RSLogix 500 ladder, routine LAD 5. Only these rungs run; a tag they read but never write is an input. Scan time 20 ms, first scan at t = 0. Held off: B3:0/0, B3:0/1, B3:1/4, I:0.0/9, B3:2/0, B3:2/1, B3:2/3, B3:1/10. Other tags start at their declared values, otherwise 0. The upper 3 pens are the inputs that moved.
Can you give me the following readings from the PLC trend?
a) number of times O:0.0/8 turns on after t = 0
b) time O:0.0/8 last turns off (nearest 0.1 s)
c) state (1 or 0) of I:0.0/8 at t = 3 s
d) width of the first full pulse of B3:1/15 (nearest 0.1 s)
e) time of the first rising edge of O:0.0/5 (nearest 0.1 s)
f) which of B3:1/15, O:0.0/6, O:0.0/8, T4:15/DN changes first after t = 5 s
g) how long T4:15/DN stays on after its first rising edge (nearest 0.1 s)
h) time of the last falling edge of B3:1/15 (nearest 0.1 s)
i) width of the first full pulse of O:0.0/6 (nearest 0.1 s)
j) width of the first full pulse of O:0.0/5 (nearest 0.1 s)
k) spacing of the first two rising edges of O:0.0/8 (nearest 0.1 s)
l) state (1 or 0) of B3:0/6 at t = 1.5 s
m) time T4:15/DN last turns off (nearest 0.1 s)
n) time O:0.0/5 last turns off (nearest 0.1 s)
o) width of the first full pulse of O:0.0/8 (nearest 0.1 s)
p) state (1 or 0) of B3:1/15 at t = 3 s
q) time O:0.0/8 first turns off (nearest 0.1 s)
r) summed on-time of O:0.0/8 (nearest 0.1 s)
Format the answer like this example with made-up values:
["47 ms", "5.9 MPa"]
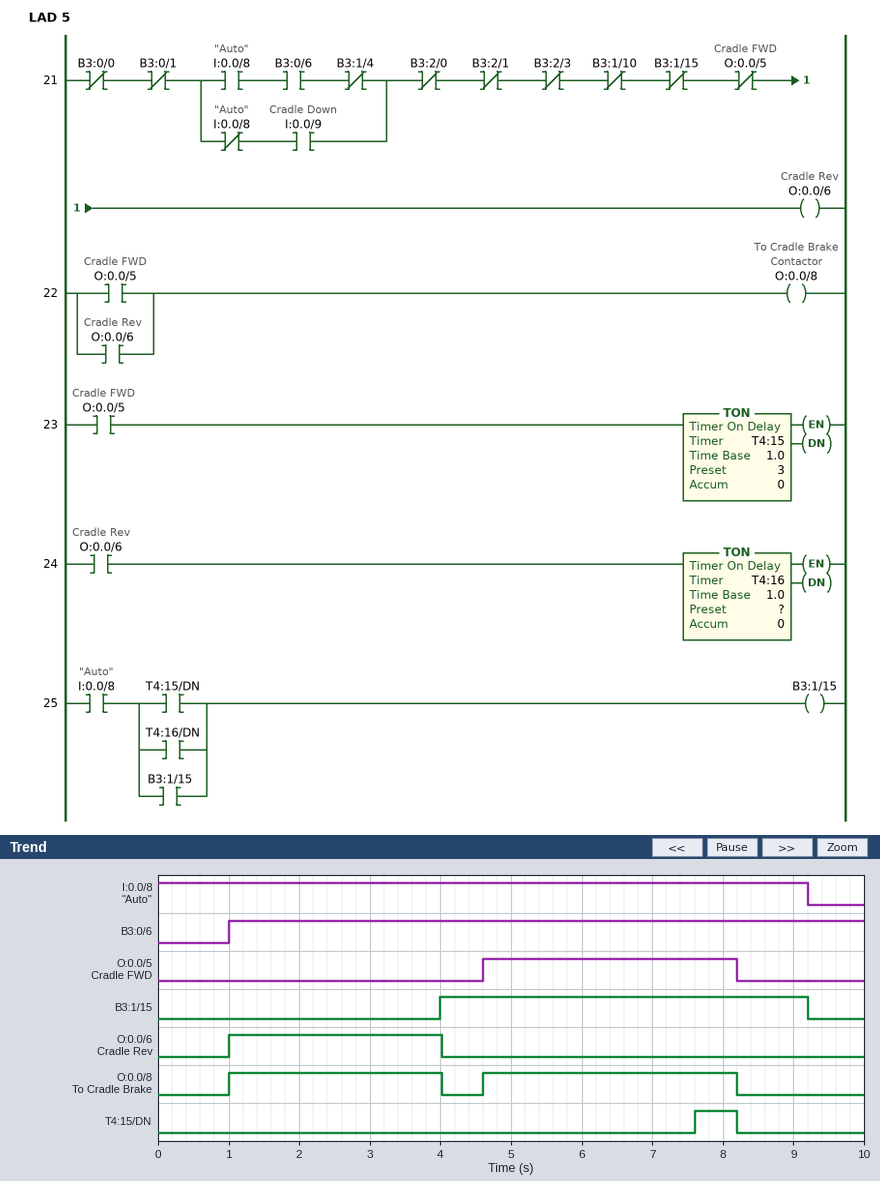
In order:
["2", "8.2 s", "1", "5.2 s", "4.6 s", "T4:15/DN", "0.6 s", "9.2 s", "3.0 s", "3.6 s", "3.6 s", "1", "8.2 s", "8.2 s", "3.0 s", "0", "4.0 s", "6.6 s"]
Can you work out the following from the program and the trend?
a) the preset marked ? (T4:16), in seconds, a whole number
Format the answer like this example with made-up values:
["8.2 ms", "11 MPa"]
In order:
["3 s"]
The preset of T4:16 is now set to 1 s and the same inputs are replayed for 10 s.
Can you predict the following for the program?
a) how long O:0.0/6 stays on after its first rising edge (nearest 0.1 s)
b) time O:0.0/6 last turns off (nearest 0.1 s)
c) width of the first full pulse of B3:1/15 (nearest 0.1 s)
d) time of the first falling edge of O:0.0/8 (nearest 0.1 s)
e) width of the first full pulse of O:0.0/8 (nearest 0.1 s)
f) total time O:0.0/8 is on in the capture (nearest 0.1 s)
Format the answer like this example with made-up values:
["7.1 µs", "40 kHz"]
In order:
["1.0 s", "2.0 s", "7.2 s", "2.0 s", "1.0 s", "4.6 s"]
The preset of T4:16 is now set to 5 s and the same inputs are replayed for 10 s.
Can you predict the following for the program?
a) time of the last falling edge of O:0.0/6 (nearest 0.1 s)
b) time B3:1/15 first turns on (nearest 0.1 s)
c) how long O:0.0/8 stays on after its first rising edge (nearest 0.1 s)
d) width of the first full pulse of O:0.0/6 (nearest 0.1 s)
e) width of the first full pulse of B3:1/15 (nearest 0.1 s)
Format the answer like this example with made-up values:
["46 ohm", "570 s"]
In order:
["4.6 s", "7.6 s", "7.2 s", "3.6 s", "1.6 s"]
